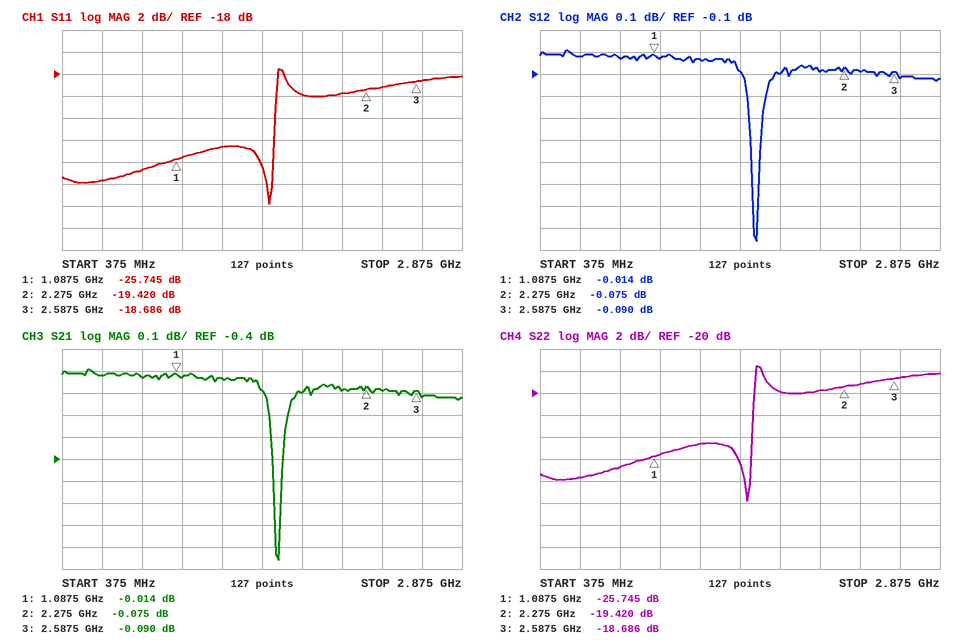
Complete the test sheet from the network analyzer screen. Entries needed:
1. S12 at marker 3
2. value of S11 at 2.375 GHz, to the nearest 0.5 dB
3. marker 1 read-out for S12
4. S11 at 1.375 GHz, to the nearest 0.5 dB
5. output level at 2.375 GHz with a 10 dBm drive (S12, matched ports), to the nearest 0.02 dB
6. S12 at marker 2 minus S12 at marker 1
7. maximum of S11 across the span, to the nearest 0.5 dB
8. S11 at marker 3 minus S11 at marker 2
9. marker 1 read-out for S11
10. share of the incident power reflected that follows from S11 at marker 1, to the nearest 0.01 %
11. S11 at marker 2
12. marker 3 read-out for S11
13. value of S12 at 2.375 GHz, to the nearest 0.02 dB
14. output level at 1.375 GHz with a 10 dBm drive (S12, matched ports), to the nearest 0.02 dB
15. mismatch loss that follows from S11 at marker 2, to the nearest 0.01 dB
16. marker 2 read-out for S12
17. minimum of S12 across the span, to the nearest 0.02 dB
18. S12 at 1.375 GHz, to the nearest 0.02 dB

-0.090 dB
-19.0 dB
-0.014 dB
-24.5 dB
9.92 dBm
-0.061 dB
-17.5 dB
0.734 dB
-25.745 dB
0.27 %
-19.420 dB
-18.686 dB
-0.08 dB
9.96 dBm
0.05 dB
-0.075 dB
-0.86 dB
-0.04 dB
